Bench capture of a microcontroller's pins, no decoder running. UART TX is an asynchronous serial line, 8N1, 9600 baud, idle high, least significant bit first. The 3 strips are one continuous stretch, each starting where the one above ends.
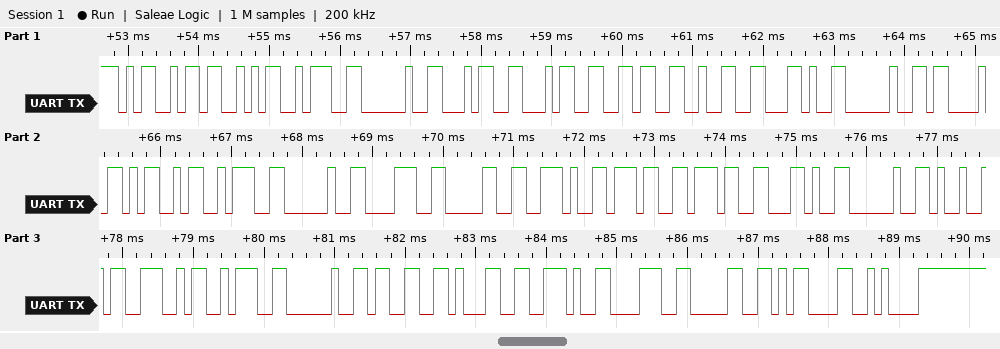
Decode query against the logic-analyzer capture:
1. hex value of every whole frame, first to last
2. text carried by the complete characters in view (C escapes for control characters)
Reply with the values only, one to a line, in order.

4D 53 3A 20 34 34 36 32 2C 20 43 4D 3A 20 38 30 2E 37 37 2C 20 49 4E 3A 20 33 31 2E 38 30 0D 0A
"MS: 4462, CM: 80.77, IN: 31.80\r\n"
